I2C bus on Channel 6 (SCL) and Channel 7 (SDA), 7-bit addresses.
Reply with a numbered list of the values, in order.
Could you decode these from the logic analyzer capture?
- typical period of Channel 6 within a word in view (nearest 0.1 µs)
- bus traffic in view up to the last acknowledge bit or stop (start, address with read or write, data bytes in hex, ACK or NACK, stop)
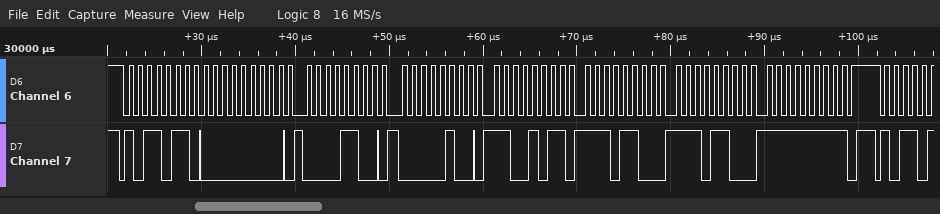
1. 1 µs
2. start, address 5B write ACK, 00 ACK, 0C ACK, 04 ACK, CB ACK, EC ACK, EC ACK, FF NACK, stop
